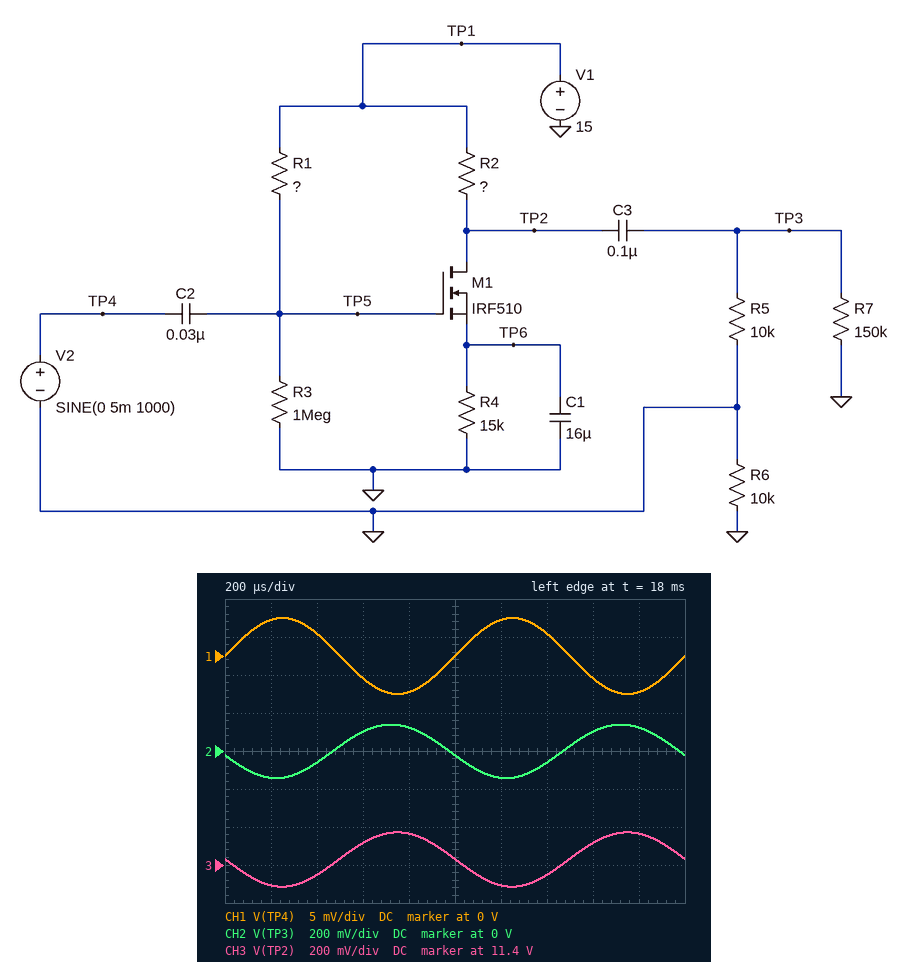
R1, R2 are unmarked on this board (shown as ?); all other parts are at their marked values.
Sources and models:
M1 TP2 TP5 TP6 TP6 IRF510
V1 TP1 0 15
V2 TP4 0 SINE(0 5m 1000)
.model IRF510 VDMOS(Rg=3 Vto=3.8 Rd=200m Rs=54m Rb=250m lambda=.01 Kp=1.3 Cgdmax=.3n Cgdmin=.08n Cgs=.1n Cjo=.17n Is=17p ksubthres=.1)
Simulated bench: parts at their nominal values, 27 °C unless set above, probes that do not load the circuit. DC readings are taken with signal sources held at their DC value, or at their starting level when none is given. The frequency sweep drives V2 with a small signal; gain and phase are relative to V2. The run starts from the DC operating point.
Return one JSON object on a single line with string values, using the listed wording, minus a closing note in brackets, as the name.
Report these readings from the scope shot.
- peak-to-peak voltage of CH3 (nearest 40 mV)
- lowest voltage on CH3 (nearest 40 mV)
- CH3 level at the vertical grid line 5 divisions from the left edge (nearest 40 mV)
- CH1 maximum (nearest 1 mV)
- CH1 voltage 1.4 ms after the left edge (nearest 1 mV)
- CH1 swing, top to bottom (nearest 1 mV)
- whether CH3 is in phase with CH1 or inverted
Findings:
{"peak-to-peak voltage of CH3": "280 mV", "lowest voltage on CH3": "11.28 V", "CH3 level at the vertical grid line 5 divisions from the left edge": "11.44 V", "CH1 maximum": "5 mV", "CH1 voltage 1.4 ms after the left edge": "3 mV", "CH1 swing, top to bottom": "10 mV", "whether CH3 is in phase with CH1 or inverted": "inverted"}
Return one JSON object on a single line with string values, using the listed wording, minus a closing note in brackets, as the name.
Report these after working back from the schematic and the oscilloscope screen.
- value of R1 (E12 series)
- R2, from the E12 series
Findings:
{"value of R1": "470 kΩ", "R2, from the E12 series": "8.2 kΩ"}
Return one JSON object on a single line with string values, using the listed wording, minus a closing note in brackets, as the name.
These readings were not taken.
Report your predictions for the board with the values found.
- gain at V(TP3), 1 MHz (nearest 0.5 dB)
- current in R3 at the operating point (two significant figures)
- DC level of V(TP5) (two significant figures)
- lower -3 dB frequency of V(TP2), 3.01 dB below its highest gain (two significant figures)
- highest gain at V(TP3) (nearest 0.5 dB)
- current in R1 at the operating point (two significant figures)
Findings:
{"gain at V(TP3), 1 MHz": "15.5 dB", "current in R3 at the operating point": "10 µA", "DC level of V(TP5)": "10 V", "lower -3 dB frequency of V(TP2), 3.01 dB below its highest gain": "38 Hz", "highest gain at V(TP3)": "29.0 dB", "current in R1 at the operating point": "10 µA"}
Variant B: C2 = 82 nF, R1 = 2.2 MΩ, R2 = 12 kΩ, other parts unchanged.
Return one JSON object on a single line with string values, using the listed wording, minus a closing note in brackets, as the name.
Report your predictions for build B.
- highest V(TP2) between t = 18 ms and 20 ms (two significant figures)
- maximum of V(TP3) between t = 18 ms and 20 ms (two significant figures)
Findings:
{"highest V(TP2) between t = 18 ms and 20 ms": "14 V", "maximum of V(TP3) between t = 18 ms and 20 ms": "36 mV"}
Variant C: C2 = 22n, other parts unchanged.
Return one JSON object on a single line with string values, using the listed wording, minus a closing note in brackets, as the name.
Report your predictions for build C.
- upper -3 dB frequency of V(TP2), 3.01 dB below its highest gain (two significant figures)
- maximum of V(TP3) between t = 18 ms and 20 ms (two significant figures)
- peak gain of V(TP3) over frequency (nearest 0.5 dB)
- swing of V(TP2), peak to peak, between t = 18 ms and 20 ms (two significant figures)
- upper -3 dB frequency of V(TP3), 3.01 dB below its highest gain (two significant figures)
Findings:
{"upper -3 dB frequency of V(TP2), 3.01 dB below its highest gain": "160 kHz", "maximum of V(TP3) between t = 18 ms and 20 ms": "130 mV", "peak gain of V(TP3) over frequency": "28.5 dB", "swing of V(TP2), peak to peak, between t = 18 ms and 20 ms": "270 mV", "upper -3 dB frequency of V(TP3), 3.01 dB below its highest gain": "220 kHz"}
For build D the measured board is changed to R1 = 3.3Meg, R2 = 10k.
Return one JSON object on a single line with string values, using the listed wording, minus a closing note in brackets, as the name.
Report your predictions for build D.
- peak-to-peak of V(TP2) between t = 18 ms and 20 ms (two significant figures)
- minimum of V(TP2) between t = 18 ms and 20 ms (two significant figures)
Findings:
{"peak-to-peak of V(TP2) between t = 18 ms and 20 ms": "4.0 mV", "minimum of V(TP2) between t = 18 ms and 20 ms": "15 V"}
